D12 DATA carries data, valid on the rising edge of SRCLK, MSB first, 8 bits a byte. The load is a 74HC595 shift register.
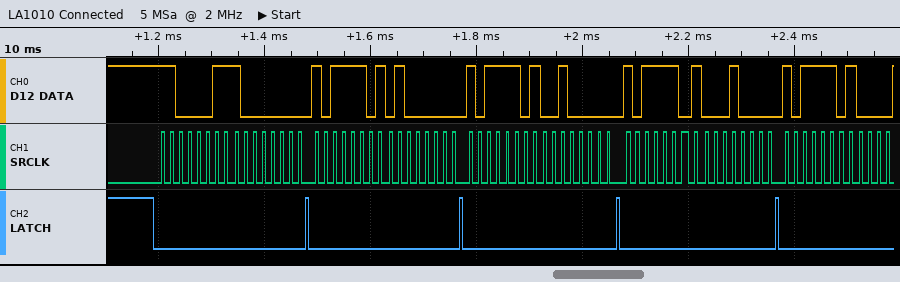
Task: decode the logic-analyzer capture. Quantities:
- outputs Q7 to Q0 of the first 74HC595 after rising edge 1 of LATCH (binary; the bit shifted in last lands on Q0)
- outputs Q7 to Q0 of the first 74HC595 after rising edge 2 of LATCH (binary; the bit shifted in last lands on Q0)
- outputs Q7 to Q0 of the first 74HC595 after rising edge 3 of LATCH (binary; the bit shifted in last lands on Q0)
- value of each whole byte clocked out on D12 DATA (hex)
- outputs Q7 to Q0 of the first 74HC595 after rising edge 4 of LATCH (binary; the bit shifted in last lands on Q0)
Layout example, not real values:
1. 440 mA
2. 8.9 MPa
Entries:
1. 10000000
2. 01000000
3. 00100000
4. C3 80 BD 40 BD 20 BD 10 BD
5. 00010000
